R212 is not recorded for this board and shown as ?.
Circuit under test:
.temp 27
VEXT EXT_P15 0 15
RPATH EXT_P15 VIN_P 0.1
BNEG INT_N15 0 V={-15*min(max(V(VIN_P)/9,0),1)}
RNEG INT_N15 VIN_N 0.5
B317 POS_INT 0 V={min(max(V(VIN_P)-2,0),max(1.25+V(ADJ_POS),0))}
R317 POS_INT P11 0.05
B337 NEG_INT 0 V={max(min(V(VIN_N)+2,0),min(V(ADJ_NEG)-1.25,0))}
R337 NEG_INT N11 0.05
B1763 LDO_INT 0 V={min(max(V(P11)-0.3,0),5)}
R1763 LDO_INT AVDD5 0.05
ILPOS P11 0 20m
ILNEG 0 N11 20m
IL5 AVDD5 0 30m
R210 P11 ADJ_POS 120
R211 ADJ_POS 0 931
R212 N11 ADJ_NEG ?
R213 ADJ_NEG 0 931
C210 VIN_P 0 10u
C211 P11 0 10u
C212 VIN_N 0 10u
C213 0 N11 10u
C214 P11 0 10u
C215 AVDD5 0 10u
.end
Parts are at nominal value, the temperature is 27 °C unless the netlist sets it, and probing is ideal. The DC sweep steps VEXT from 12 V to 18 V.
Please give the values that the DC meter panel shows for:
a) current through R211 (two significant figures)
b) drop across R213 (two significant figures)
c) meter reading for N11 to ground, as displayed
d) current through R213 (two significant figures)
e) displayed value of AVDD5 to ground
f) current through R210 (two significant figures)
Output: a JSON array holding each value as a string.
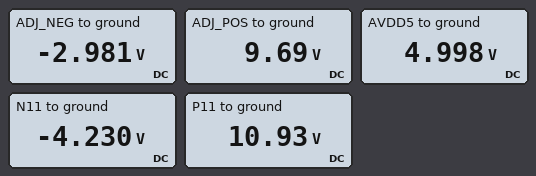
["10 mA", "3.0 V", "-4.230 V", "3.2 mA", "4.998 V", "10 mA"]
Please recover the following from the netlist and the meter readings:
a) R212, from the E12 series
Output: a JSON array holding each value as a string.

["390 Ω"]
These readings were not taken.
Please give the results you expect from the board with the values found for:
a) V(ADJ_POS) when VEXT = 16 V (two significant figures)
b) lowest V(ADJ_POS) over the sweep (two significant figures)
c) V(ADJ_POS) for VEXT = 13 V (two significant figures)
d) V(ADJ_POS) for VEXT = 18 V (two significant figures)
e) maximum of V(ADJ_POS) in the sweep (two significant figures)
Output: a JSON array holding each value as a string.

["9.7 V", "8.9 V", "9.7 V", "9.7 V", "9.7 V"]
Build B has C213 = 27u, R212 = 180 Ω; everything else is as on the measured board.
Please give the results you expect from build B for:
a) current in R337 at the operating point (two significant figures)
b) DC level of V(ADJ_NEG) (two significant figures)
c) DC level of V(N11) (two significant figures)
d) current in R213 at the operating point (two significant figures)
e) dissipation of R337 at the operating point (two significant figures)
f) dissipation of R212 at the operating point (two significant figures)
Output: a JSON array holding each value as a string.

["27 mA", "-6.5 V", "-7.7 V", "6.9 mA", "36 µW", "8.7 mW"]
